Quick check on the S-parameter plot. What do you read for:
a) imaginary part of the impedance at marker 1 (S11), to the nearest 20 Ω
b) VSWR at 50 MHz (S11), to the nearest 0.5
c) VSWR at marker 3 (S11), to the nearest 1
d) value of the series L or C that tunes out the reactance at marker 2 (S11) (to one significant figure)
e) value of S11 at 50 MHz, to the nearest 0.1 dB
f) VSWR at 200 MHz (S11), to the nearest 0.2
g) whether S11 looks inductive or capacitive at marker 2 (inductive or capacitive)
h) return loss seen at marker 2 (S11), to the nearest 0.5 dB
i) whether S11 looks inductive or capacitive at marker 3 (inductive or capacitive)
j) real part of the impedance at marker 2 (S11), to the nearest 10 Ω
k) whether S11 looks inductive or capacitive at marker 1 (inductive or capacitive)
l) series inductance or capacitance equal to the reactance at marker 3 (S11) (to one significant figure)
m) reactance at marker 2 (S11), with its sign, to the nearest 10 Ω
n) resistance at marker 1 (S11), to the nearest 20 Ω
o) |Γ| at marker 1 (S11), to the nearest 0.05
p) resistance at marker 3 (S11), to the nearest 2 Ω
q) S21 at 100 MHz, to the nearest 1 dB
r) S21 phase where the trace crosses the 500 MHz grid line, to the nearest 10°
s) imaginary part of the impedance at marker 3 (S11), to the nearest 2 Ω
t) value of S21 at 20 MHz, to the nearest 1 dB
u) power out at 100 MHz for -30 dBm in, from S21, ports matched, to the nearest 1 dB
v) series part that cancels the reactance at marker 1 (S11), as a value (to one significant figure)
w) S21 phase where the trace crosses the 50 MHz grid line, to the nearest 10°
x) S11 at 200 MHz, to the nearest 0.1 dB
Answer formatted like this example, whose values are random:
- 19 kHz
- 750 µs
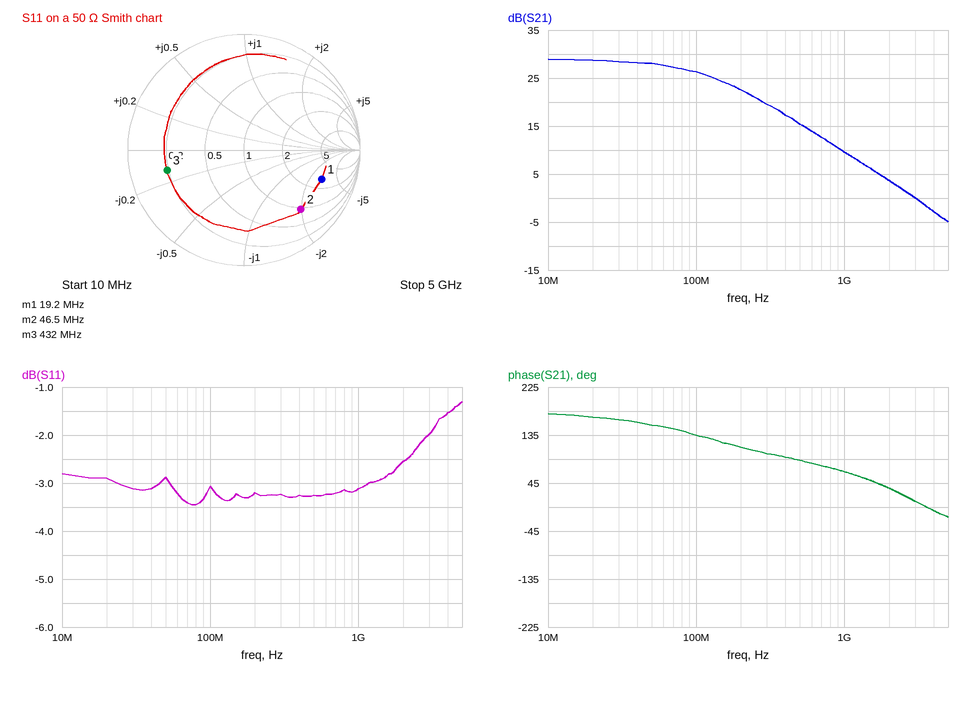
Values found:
- -140 Ω
- 6.0
- 5
- 300 nH
- -2.9 dB
- 5.4
- capacitive
- 3.0 dB
- capacitive
- 50 Ω
- capacitive
- 60 pF
- -100 Ω
- 140 Ω
- 0.70
- 10 Ω
- 26 dB
- 90°
- -6 Ω
- 29 dB
- -4 dBm
- 1 µH
- 150°
- -3.2 dB
